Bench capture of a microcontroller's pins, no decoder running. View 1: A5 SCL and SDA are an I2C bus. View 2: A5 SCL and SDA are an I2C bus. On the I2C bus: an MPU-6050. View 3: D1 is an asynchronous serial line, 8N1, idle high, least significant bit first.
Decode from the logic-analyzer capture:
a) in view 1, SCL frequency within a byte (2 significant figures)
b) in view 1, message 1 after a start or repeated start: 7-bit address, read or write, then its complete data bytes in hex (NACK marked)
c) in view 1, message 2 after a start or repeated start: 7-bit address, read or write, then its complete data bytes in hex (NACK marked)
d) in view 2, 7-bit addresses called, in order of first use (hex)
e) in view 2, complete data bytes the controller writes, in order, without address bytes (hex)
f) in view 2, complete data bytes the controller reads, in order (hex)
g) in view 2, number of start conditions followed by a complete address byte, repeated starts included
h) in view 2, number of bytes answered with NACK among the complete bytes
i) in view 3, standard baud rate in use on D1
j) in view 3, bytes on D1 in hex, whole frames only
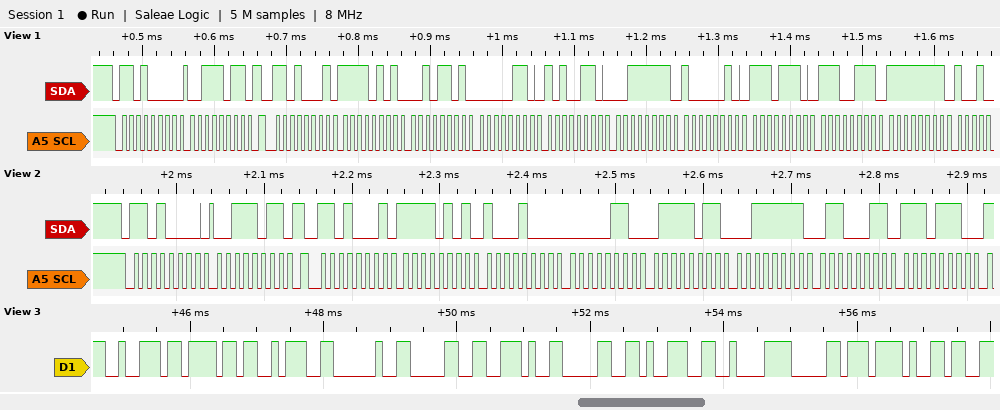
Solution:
100 kHz
0x68 write: 3B
0x68 read: F5 2D 06 A6 3F 82 EE E7 FF
0x68
3B
F5 88 06 7B 3F 63 EE
2
0
9600 baud
72 6F 3A 20 30 2E 30 39 C2 B0 2F
